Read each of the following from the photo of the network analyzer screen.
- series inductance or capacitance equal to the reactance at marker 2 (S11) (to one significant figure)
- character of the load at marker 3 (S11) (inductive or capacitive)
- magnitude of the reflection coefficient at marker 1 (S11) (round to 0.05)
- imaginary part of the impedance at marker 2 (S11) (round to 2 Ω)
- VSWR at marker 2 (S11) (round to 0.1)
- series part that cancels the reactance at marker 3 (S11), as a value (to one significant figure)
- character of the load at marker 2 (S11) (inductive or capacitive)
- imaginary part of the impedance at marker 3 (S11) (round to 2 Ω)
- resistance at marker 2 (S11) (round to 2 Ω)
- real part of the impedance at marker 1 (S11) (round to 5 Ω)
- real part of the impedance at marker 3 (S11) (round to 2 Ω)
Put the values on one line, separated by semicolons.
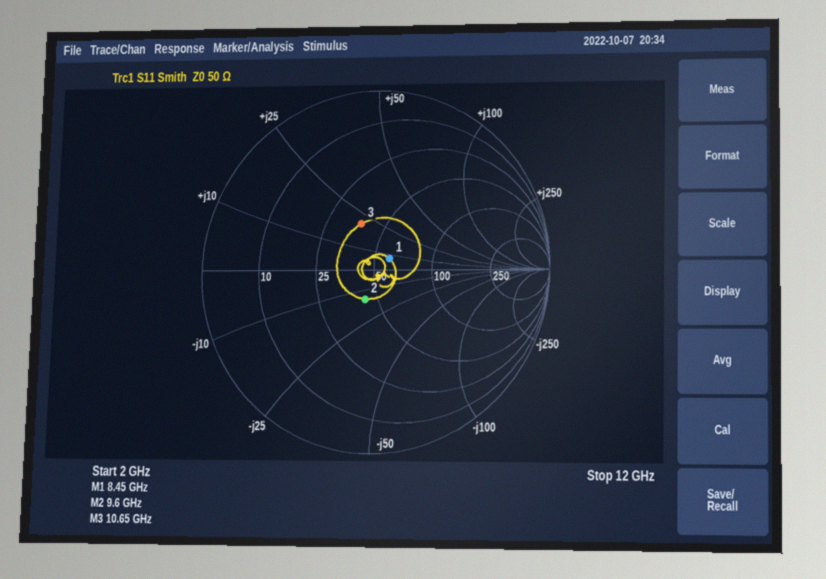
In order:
1 pF; inductive; 0.10; -14 Ω; 1.4; 700 fF; capacitive; +20 Ω; 44 Ω; 60 Ω; 38 Ω
